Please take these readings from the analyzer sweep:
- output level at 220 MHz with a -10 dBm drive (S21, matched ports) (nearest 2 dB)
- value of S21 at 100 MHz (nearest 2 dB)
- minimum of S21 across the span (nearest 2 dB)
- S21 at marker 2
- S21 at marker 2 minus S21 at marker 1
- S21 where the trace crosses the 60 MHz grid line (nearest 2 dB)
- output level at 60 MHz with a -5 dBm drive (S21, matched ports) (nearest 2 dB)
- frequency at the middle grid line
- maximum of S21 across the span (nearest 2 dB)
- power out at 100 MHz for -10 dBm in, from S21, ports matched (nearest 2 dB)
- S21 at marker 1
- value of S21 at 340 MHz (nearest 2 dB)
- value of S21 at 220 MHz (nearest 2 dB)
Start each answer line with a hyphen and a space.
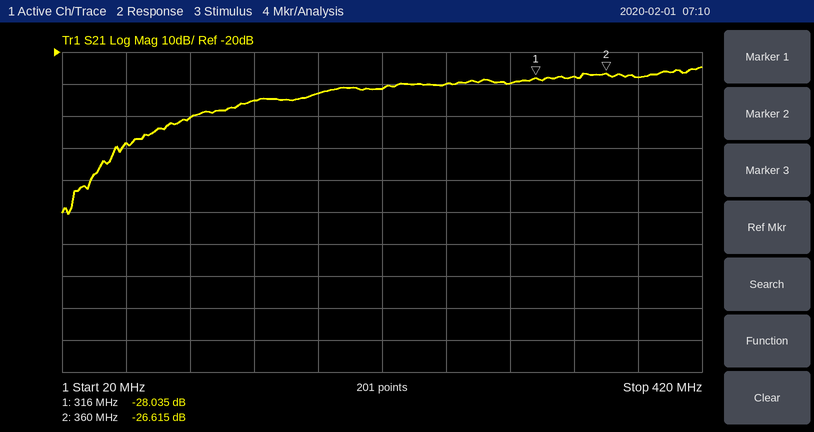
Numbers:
- -42 dBm
- -40 dB
- -70 dB
- -26.615 dB
- 1.420 dB
- -48 dB
- -54 dBm
- 220 MHz
- -24 dB
- -50 dBm
- -28.035 dB
- -28 dB
- -32 dB
